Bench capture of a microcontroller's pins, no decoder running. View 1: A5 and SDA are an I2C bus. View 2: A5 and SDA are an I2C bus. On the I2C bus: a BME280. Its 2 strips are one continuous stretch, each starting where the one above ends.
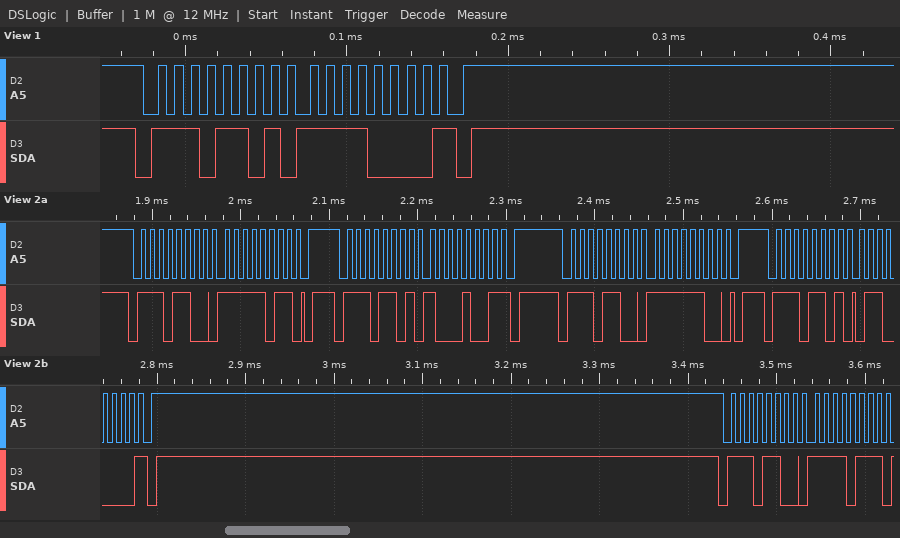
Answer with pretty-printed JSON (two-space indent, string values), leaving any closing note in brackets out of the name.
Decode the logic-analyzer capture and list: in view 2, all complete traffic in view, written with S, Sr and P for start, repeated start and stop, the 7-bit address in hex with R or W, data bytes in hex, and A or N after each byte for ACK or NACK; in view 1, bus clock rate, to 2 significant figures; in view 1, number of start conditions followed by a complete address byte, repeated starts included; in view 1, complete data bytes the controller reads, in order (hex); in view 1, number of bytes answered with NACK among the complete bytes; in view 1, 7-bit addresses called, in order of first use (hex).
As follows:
{
  "in view 2, all complete traffic in view, written with S, Sr and P for start, repeated start and stop, the 7-bit address in hex with R or W, data bytes in hex, and A or N after each byte for ACK or NACK": "S 76W A FB A P S 76R A 89 N P S 76W A FC A P S 76R A 60 N P S 76W A F7 A",
  "in view 1, bus clock rate, to 2 significant figures": "100 kHz",
  "in view 1, number of start conditions followed by a complete address byte, repeated starts included": "1",
  "in view 1, complete data bytes the controller reads, in order": "F0",
  "in view 1, number of bytes answered with NACK among the complete bytes": "1",
  "in view 1, 7-bit addresses called, in order of first use": "0x76"
}
